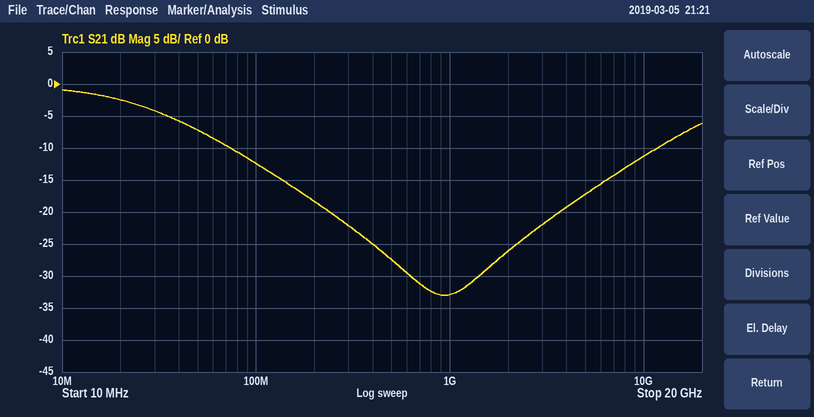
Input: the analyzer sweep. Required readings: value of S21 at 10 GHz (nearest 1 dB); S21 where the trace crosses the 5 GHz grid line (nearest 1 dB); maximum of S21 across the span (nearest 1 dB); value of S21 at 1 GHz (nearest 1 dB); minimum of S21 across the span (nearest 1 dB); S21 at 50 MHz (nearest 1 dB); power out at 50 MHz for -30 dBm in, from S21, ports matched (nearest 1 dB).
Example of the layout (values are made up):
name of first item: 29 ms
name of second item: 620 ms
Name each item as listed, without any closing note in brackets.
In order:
value of S21 at 10 GHz: -11 dB
S21 where the trace crosses the 5 GHz grid line: -17 dB
maximum of S21 across the span: -1 dB
value of S21 at 1 GHz: -33 dB
minimum of S21 across the span: -33 dB
S21 at 50 MHz: -7 dB
power out at 50 MHz for -30 dBm in, from S21, ports matched: -37 dBm
